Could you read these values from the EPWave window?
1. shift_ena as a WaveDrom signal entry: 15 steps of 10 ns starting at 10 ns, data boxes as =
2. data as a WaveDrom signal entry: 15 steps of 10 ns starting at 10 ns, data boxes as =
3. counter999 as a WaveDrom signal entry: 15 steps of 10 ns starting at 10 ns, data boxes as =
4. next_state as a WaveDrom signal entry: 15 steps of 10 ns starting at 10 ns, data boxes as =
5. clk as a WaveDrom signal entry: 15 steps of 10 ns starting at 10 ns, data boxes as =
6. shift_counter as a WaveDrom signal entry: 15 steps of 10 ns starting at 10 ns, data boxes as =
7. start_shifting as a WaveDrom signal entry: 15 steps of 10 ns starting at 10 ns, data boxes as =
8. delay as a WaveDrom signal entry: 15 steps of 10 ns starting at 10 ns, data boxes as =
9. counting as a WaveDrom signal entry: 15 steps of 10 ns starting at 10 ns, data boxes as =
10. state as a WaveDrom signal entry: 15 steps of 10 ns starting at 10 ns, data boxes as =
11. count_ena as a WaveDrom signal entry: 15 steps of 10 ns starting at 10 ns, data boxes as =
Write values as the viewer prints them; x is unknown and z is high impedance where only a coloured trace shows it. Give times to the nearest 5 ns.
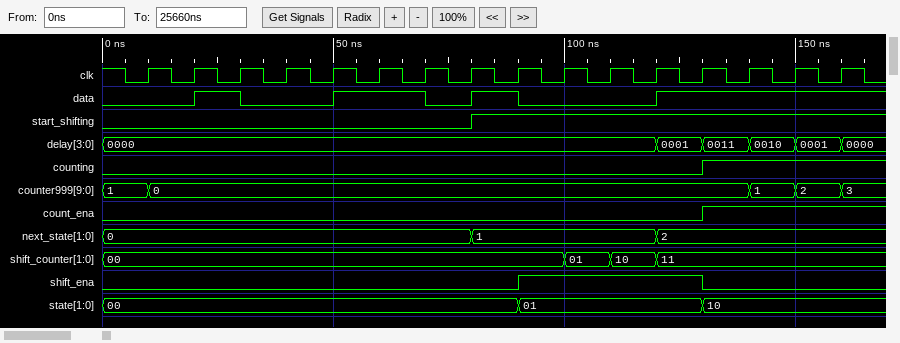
{name: 'shift_ena', wave: '0.......1...0..'}
{name: 'data', wave: '010.1.010..1...'}
{name: 'counter999', wave: '=............==', data: '0 1 2'}
{name: 'next_state', wave: '=......=...=...', data: '0 1 2'}
{name: 'clk', wave: 'p..............'}
{name: 'shift_counter', wave: '=........===...', data: '00 01 10 11'}
{name: 'start_shifting', wave: '0......1.......'}
{name: 'delay', wave: '=..........====', data: '0000 0001 0011 0010 0001'}
{name: 'counting', wave: '0...........1..'}
{name: 'state', wave: '=.......=...=..', data: '00 01 10'}
{name: 'count_ena', wave: '0...........1..'}
